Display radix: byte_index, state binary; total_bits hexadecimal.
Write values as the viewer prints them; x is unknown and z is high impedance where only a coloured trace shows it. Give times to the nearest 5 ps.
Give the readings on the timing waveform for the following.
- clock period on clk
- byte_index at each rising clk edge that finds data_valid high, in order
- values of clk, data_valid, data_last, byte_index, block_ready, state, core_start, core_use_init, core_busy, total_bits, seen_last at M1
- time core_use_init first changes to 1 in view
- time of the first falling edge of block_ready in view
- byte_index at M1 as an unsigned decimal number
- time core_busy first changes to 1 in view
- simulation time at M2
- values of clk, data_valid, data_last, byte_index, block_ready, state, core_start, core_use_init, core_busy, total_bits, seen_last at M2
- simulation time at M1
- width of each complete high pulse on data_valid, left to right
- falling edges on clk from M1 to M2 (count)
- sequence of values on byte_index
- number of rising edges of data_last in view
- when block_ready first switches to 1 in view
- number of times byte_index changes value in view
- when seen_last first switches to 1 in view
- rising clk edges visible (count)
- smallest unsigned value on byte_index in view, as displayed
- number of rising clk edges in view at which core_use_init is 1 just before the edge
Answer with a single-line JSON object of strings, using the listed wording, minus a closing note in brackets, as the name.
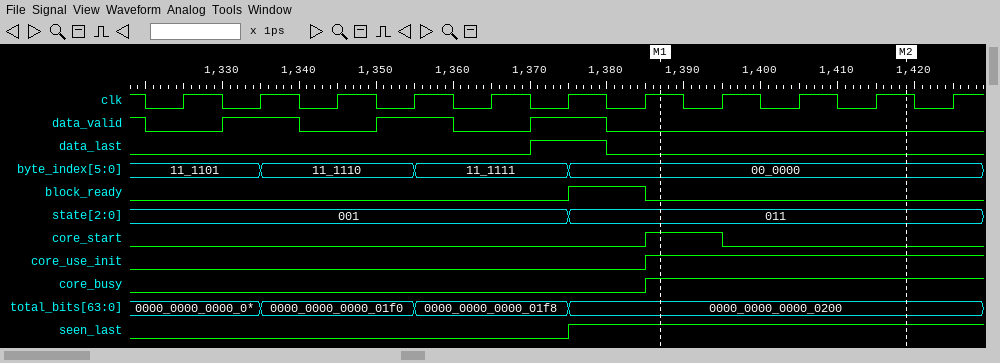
{"clock period on clk": "10 ps", "byte_index at each rising clk edge that finds data_valid high, in order": "11_1101, 11_1110, 11_1111", "values of clk, data_valid, data_last, byte_index, block_ready, state, core_start, core_use_init, core_busy, total_bits, seen_last at M1": "clk=1, data_valid=0, data_last=0, byte_index=00_0000, block_ready=0, state=011, core_start=1, core_use_init=1, core_busy=1, total_bits=0000_0000_0000_0200, seen_last=1", "time core_use_init first changes to 1 in view": "1385 ps", "time of the first falling edge of block_ready in view": "1385 ps", "byte_index at M1 as an unsigned decimal number": "0", "time core_busy first changes to 1 in view": "1385 ps", "simulation time at M2": "1420 ps", "values of clk, data_valid, data_last, byte_index, block_ready, state, core_start, core_use_init, core_busy, total_bits, seen_last at M2": "clk=1, data_valid=0, data_last=0, byte_index=00_0000, block_ready=0, state=011, core_start=0, core_use_init=1, core_busy=1, total_bits=0000_0000_0000_0200, seen_last=1", "simulation time at M1": "1385 ps", "width of each complete high pulse on data_valid, left to right": "10 ps, 10 ps, 10 ps", "falling edges on clk from M1 to M2": "3", "sequence of values on byte_index": "11_1101, 11_1110, 11_1111, 00_0000", "number of rising edges of data_last in view": "1", "when block_ready first switches to 1 in view": "1375 ps", "number of times byte_index changes value in view": "3", "when seen_last first switches to 1 in view": "1375 ps", "rising clk edges visible": "11", "smallest unsigned value on byte_index in view, as displayed": "00_0000", "number of rising clk edges in view at which core_use_init is 1 just before the edge": "4"}
